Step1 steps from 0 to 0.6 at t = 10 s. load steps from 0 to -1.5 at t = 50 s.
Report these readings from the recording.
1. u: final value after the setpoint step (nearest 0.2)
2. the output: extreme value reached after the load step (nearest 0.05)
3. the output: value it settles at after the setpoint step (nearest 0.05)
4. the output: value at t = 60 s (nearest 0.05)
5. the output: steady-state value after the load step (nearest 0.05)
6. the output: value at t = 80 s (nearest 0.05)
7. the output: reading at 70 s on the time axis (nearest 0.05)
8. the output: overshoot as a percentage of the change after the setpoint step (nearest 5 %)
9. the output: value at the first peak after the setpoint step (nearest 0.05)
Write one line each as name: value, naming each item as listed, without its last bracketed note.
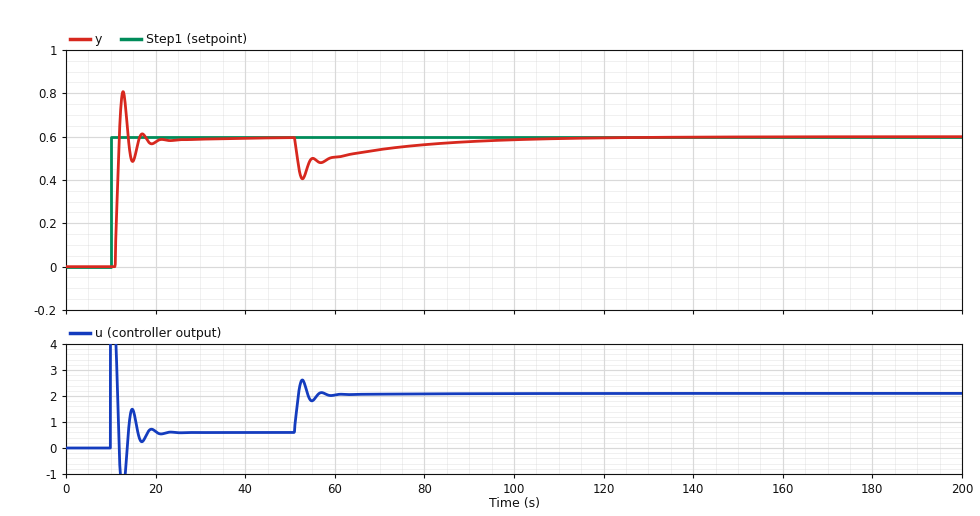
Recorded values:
u: final value after the setpoint step: 0.6
the output: extreme value reached after the load step: 0.40
the output: value it settles at after the setpoint step: 0.60
the output: value at t = 60 s: 0.50
the output: steady-state value after the load step: 0.60
the output: value at t = 80 s: 0.55
the output: reading at 70 s on the time axis: 0.55
the output: overshoot as a percentage of the change after the setpoint step: 35 %
the output: value at the first peak after the setpoint step: 0.80
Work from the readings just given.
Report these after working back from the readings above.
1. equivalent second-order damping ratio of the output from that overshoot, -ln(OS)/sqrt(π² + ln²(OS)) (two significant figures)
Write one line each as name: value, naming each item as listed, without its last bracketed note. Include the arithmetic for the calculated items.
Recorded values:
equivalent second-order damping ratio of the output from that overshoot, -ln(OS)/sqrt(π² + ln²(OS)): ln(0.35) = -1.050; 1.050 / sqrt(9.870 + 1.102) = 0.32
